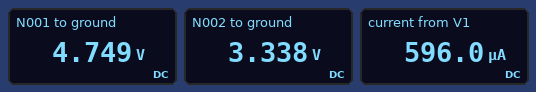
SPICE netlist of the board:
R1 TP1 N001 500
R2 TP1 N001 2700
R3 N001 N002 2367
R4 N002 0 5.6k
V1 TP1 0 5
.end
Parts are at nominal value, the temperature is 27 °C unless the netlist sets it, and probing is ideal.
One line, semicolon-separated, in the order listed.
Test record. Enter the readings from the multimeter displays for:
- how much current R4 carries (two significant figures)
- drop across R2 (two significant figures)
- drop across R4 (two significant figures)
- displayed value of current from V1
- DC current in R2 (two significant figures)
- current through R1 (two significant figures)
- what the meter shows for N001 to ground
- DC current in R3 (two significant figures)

600 µA; 250 mV; 3.3 V; 596.0 µA; 93 µA; 500 µA; 4.749 V; 600 µA
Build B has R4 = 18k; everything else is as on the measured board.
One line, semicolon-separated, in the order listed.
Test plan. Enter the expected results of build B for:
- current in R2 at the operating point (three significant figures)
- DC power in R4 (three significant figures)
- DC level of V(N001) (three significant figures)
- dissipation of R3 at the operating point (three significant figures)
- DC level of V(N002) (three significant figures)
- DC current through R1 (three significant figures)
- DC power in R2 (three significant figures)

37.6 µA; 1.04 mW; 4.90 V; 137 µW; 4.33 V; 203 µA; 3.81 µW
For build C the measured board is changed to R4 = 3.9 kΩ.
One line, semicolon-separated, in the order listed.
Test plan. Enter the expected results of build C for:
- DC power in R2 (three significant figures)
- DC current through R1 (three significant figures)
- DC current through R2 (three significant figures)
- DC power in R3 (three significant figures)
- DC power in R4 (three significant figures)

36.8 µW; 631 µA; 117 µA; 1.32 mW; 2.18 mW
